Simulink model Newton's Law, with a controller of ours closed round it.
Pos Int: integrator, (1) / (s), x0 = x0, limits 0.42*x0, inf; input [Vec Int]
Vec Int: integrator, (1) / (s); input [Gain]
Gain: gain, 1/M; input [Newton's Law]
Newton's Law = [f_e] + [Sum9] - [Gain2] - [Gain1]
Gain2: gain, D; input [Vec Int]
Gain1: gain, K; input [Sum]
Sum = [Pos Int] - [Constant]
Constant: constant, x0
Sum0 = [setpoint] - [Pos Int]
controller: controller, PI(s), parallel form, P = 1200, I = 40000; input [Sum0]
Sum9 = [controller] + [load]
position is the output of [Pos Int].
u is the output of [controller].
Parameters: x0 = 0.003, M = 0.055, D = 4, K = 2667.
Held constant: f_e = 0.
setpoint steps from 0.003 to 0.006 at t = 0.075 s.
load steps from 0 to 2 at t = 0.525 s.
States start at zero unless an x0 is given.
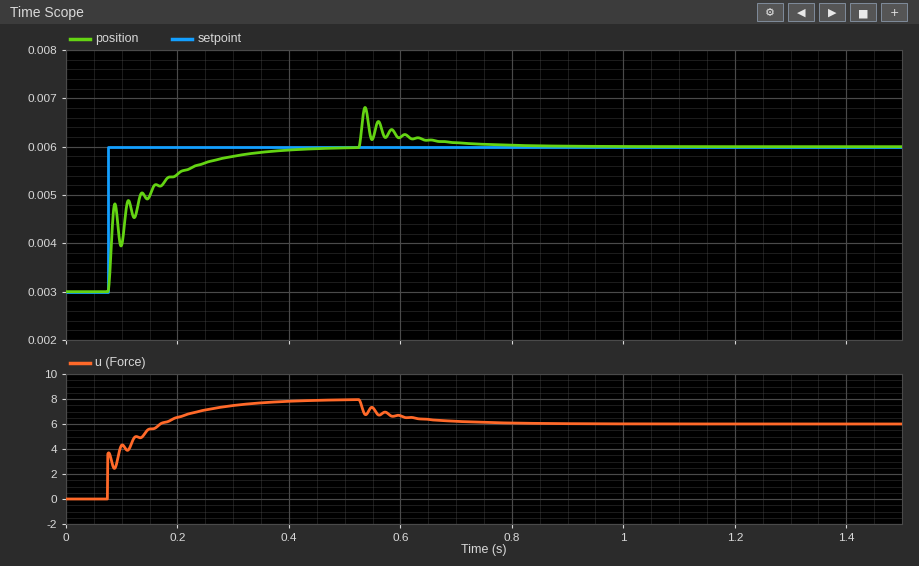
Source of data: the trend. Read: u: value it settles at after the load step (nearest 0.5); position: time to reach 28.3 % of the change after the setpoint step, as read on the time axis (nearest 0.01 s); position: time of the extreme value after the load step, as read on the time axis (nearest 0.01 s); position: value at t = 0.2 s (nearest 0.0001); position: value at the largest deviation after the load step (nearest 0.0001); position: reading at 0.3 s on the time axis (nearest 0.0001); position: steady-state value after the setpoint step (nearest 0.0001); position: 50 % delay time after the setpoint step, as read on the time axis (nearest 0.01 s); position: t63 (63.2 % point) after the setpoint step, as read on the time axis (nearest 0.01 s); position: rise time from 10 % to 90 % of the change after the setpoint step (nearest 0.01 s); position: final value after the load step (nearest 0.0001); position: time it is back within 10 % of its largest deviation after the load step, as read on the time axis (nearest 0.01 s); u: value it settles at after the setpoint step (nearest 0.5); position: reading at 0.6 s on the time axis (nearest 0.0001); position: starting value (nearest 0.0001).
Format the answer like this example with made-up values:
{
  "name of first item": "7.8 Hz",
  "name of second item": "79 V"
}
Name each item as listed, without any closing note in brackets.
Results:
{
  "u: value it settles at after the load step": "6.0",
  "position: time to reach 28.3 % of the change after the setpoint step, as read on the time axis": "0.08 s",
  "position: time of the extreme value after the load step, as read on the time axis": "0.54 s",
  "position: value at t = 0.2 s": "0.0054",
  "position: value at the largest deviation after the load step": "0.0068",
  "position: reading at 0.3 s on the time axis": "0.0058",
  "position: steady-state value after the setpoint step": "0.0060",
  "position: 50 % delay time after the setpoint step, as read on the time axis": "0.08 s",
  "position: t63 (63.2 % point) after the setpoint step, as read on the time axis": "0.13 s",
  "position: rise time from 10 % to 90 % of the change after the setpoint step": "0.18 s",
  "position: final value after the load step": "0.0060",
  "position: time it is back within 10 % of its largest deviation after the load step, as read on the time axis": "0.70 s",
  "u: value it settles at after the setpoint step": "8.0",
  "position: reading at 0.6 s on the time axis": "0.0062",
  "position: starting value": "0.0030"
}
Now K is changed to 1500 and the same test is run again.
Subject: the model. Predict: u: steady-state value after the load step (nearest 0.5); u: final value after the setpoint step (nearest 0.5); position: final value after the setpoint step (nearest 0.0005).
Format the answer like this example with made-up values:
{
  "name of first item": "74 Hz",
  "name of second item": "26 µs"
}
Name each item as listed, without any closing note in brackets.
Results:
{
  "u: steady-state value after the load step": "2.5",
  "u: final value after the setpoint step": "4.5",
  "position: final value after the setpoint step": "0.0060"
}
